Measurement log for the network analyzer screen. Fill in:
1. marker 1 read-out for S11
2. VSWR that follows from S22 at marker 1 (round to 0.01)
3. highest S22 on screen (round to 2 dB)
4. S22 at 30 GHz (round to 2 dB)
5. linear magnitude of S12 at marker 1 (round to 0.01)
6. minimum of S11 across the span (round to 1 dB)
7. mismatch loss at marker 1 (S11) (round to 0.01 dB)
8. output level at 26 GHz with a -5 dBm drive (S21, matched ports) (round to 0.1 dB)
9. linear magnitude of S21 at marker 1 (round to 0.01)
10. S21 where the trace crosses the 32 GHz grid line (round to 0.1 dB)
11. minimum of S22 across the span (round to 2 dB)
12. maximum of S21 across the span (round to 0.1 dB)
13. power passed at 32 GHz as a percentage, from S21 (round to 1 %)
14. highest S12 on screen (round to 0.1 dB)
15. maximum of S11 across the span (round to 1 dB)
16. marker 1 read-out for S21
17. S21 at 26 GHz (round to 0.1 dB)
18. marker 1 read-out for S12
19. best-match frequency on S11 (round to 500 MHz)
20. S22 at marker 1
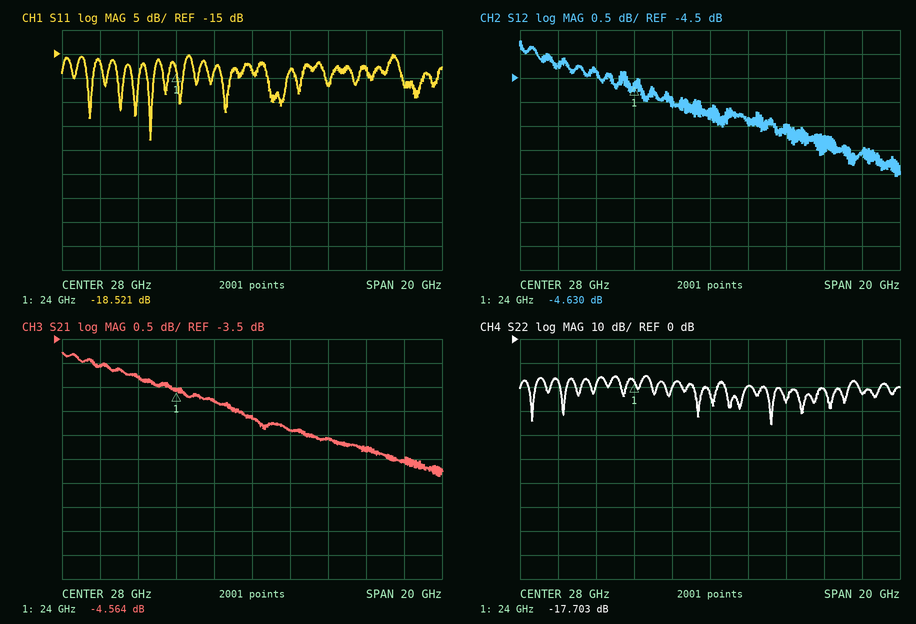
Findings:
-18.521 dB
1.30
-16 dB
-20 dB
0.59
-33 dB
0.06 dB
-9.8 dBm
0.59
-5.6 dB
-36 dB
-3.8 dB
28 %
-3.7 dB
-15 dB
-4.564 dB
-4.8 dB
-4.630 dB
22.5 GHz
-17.703 dB
